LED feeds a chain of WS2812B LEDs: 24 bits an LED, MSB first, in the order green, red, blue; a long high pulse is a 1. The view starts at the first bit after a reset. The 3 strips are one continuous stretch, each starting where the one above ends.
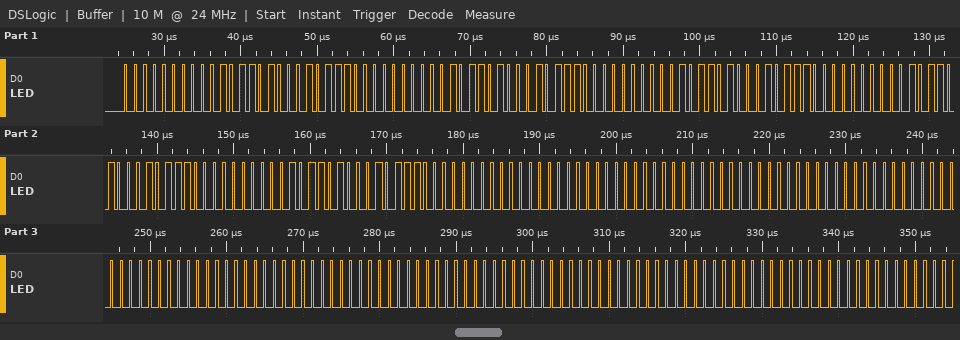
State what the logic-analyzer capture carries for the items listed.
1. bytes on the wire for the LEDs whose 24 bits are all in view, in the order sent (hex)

00 2D 17 00 2D 17 00 2D 17 00 2D 17 00 2D 17 00 00 00 00 00 00 00 00 00 00 00 00 00 00 00 00 00 00
